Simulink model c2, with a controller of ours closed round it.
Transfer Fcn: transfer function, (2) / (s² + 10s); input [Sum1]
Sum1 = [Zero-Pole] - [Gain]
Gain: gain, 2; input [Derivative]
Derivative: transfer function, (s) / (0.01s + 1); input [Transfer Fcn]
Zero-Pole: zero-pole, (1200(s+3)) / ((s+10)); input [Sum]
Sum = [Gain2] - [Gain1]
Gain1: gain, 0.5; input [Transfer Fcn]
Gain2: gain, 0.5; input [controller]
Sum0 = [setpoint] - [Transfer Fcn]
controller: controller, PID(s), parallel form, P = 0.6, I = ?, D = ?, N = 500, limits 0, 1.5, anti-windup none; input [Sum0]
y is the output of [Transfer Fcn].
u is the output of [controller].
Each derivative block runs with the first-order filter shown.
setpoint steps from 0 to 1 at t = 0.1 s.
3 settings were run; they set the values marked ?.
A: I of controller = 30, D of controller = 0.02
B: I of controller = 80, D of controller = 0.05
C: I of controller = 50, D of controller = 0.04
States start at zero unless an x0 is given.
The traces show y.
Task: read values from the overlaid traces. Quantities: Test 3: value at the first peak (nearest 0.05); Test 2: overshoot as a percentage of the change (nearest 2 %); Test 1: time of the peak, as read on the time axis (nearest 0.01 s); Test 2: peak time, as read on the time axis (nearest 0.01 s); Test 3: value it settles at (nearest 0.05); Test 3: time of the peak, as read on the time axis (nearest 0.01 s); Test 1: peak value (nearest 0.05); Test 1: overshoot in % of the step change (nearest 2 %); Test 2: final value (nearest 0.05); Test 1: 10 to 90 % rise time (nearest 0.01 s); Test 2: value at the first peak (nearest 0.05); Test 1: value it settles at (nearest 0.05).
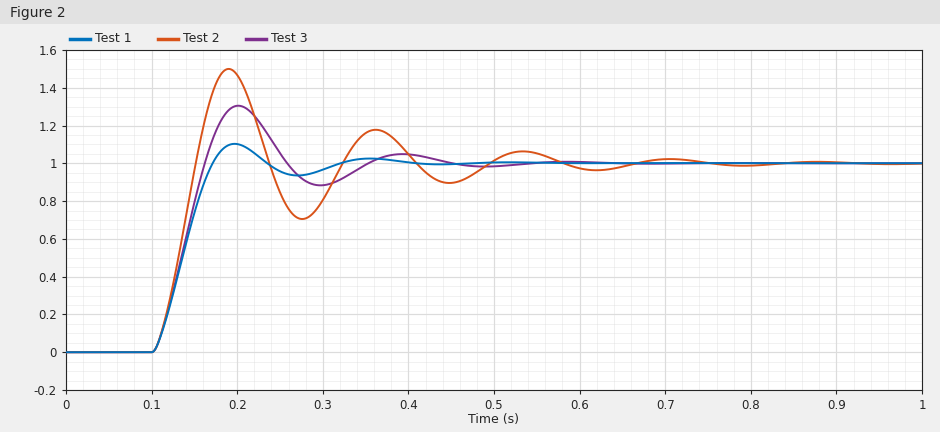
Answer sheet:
1.30
50 %
0.20 s
0.19 s
1.00
0.20 s
1.10
10 %
1.00
0.05 s
1.50
1.00
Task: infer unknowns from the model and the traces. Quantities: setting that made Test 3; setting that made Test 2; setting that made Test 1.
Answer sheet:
C
B
A
